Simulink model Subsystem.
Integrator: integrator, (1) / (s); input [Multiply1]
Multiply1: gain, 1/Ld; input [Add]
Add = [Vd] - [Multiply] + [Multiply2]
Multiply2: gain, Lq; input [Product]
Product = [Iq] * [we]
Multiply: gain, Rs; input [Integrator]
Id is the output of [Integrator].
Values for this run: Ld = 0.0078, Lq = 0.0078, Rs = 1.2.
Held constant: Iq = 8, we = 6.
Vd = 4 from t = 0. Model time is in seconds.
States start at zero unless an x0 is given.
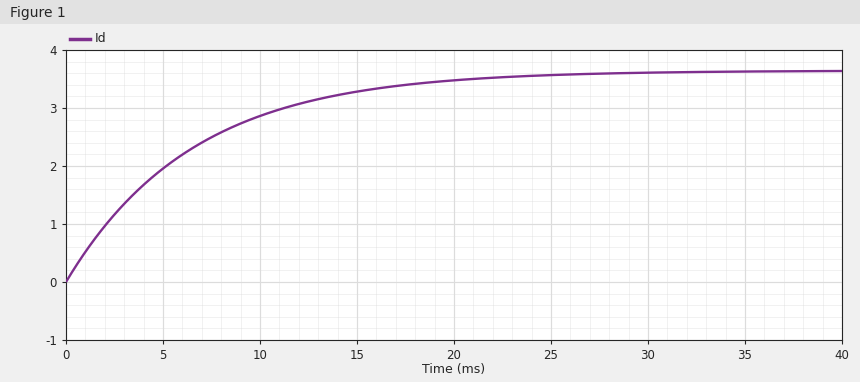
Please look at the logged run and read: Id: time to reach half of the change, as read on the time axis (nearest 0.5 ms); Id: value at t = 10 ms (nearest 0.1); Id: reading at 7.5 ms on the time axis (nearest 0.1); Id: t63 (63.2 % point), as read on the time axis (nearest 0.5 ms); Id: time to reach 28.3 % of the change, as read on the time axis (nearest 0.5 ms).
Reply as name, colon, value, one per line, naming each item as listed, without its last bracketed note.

Id: time to reach half of the change, as read on the time axis: 4.5 ms
Id: value at t = 10 ms: 2.9
Id: reading at 7.5 ms on the time axis: 2.5
Id: t63 (63.2 % point), as read on the time axis: 6.5 ms
Id: time to reach 28.3 % of the change, as read on the time axis: 2.0 ms
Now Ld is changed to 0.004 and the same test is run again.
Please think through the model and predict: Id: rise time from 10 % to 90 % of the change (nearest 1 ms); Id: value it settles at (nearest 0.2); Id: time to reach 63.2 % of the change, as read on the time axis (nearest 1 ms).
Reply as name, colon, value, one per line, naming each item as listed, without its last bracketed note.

Id: rise time from 10 % to 90 % of the change: 7 ms
Id: value it settles at: 3.6
Id: time to reach 63.2 % of the change, as read on the time axis: 3 ms
